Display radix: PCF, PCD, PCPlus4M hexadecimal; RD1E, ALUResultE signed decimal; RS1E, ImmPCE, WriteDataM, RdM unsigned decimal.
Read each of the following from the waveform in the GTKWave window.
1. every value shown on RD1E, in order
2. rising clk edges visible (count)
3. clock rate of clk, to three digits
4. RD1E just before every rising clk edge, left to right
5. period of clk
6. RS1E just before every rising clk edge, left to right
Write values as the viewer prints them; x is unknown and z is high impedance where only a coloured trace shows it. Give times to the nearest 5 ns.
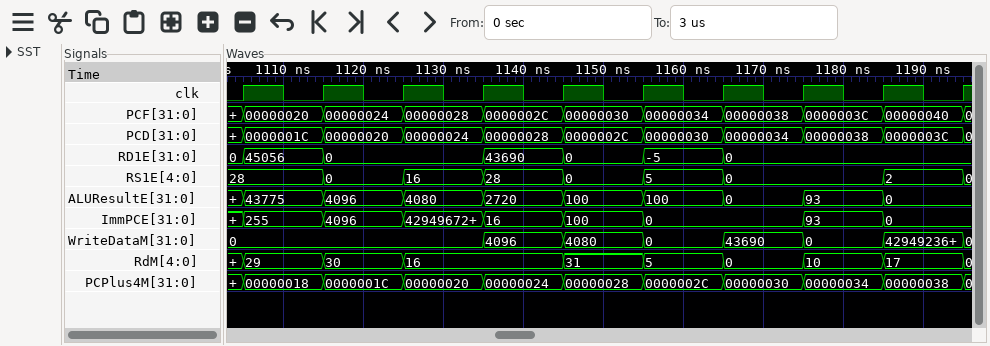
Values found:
0, 45056, 0, 43690, 0, -5, 0
10
100 MHz
0, 45056, 0, 0, 43690, 0, -5, 0, 0, 0
10 ns
28, 28, 0, 16, 28, 0, 5, 0, 0, 2
